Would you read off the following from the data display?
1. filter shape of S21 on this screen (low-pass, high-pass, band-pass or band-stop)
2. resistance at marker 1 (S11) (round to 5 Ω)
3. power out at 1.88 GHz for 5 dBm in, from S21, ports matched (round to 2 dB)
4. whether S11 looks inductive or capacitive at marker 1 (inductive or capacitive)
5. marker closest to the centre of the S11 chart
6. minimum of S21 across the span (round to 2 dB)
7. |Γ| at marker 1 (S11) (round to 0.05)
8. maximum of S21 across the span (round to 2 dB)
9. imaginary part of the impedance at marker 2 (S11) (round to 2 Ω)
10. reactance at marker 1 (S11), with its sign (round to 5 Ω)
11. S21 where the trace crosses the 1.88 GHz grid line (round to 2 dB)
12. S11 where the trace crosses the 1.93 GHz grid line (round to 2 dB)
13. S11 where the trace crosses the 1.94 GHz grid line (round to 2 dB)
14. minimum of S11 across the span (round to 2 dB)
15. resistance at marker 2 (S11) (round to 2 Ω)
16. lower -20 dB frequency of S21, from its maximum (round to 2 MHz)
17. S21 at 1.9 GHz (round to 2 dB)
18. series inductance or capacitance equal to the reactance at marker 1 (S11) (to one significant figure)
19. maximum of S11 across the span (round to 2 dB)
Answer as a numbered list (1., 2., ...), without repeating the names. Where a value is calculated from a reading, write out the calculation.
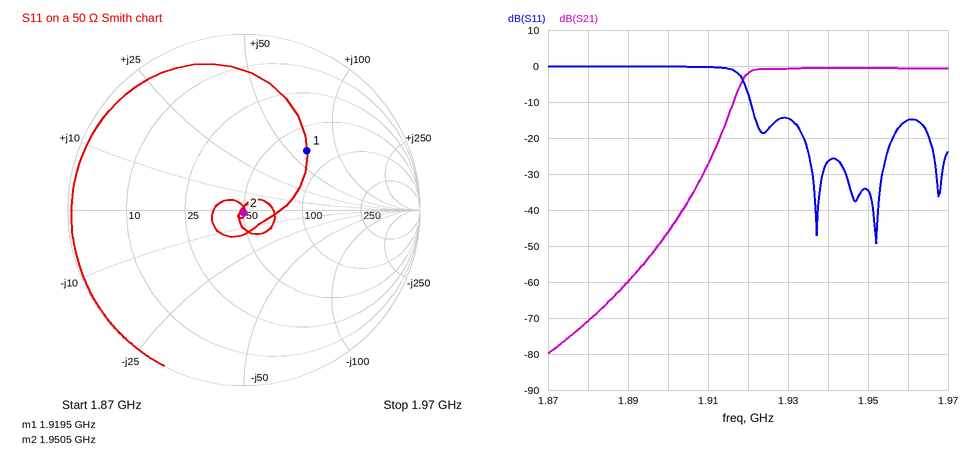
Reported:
1. high-pass
2. 70 Ω
3. 5 dBm + (-70 dB) = -66 dBm
4. inductive
5. marker 2
6. -80 dB
7. 0.50
8. 0 dB
9. -2 Ω
10. +65 Ω
11. -70 dB
12. -14 dB
13. -26 dB
14. -50 dB
15. 50 Ω
16. 1.912 GHz
17. -46 dB
18. L = 65 Ω/(2π × 1.9195 GHz) ≈ 5 nH
19. 0 dB
